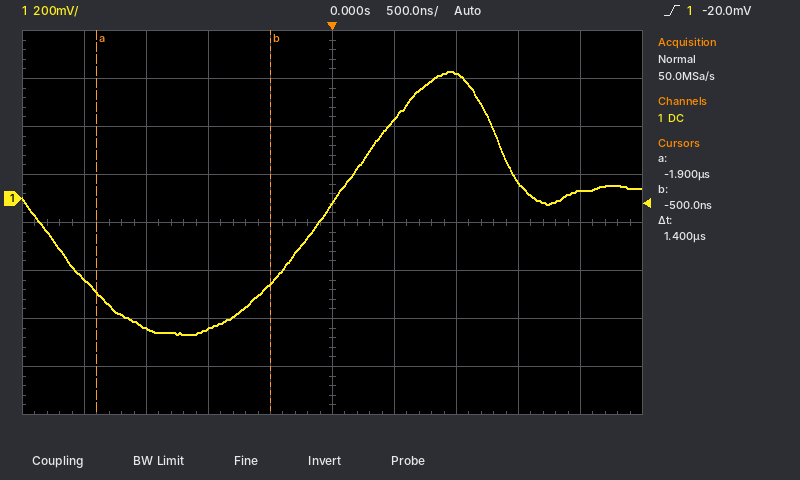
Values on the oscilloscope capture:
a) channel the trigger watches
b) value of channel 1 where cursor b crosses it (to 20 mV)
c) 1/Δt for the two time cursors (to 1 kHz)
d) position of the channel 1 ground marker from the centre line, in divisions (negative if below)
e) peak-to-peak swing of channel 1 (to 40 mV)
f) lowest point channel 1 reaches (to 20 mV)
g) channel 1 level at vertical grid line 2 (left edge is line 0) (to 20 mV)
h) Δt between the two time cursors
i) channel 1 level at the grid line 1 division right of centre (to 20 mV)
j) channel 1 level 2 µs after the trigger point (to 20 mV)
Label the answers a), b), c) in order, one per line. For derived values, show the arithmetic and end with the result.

a) channel 1
b) -360 mV
c) 1 / 1.4 µs ≈ 714 kHz
d) +0.5 div
e) 1.08 V
f) -560 mV
g) -540 mV
h) 1.4 µs
i) 320 mV
j) 40 mV
